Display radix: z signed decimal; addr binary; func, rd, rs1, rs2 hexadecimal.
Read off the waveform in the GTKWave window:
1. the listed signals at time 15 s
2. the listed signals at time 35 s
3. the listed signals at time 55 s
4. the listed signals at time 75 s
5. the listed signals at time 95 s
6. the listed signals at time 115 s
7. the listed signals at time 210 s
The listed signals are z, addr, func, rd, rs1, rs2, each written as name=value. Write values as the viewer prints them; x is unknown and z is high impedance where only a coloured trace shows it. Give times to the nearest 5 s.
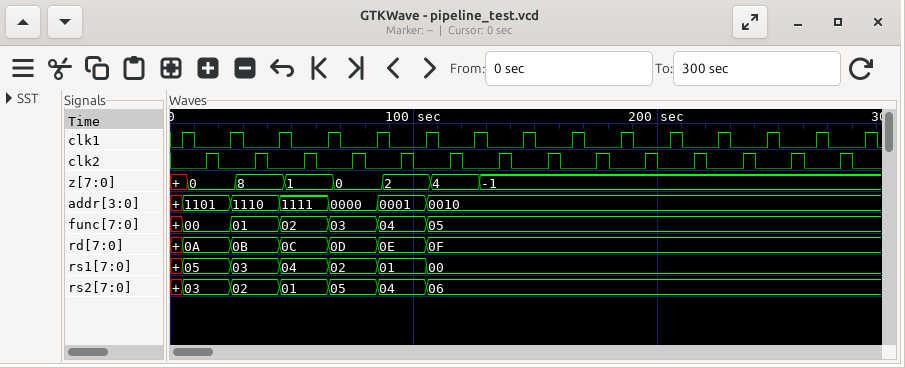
z=0, addr=1101, func=00, rd=0A, rs1=05, rs2=03
z=8, addr=1110, func=01, rd=0B, rs1=03, rs2=02
z=1, addr=1111, func=02, rd=0C, rs1=04, rs2=01
z=0, addr=0000, func=03, rd=0D, rs1=02, rs2=05
z=2, addr=0001, func=04, rd=0E, rs1=01, rs2=04
z=4, addr=0010, func=05, rd=0F, rs1=00, rs2=06
z=-1, addr=0010, func=05, rd=0F, rs1=00, rs2=06
